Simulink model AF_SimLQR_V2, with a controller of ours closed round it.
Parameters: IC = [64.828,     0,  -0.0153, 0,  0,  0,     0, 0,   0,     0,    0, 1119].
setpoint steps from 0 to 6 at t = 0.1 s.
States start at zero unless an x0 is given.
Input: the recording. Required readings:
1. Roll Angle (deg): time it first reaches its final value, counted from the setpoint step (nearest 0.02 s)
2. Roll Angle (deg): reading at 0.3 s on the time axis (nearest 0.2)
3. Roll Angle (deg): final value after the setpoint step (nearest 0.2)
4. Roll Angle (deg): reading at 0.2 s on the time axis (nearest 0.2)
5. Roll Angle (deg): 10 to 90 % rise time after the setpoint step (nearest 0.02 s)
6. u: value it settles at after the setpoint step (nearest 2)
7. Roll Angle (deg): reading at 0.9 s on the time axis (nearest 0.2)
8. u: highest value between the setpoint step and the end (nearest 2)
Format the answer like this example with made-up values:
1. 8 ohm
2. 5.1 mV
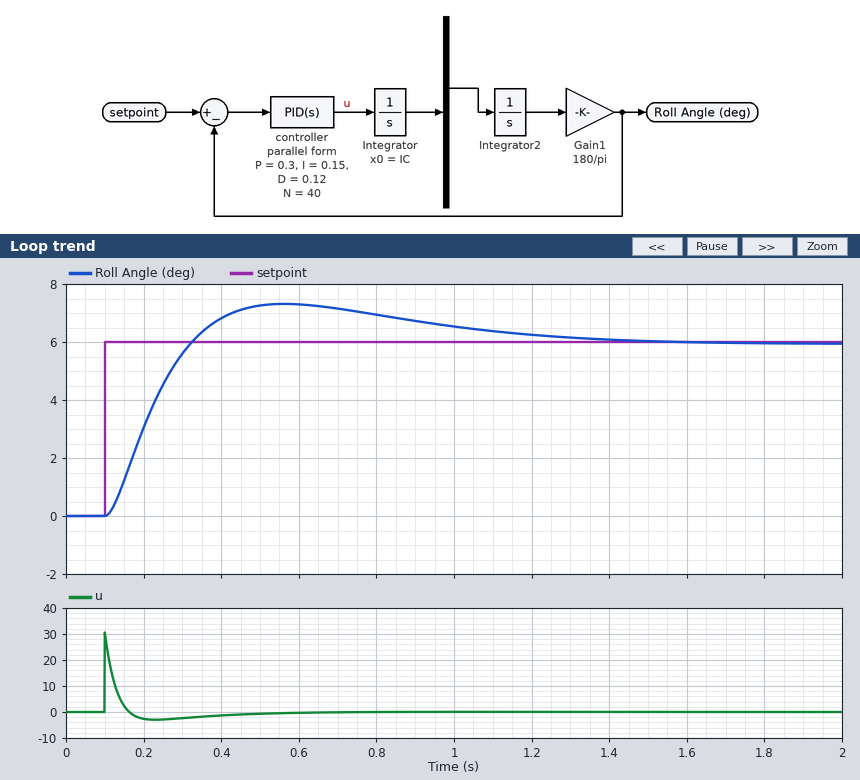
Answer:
1. 0.22 s
2. 5.6
3. 6.0
4. 3.0
5. 0.16 s
6. 0
7. 6.8
8. 30
